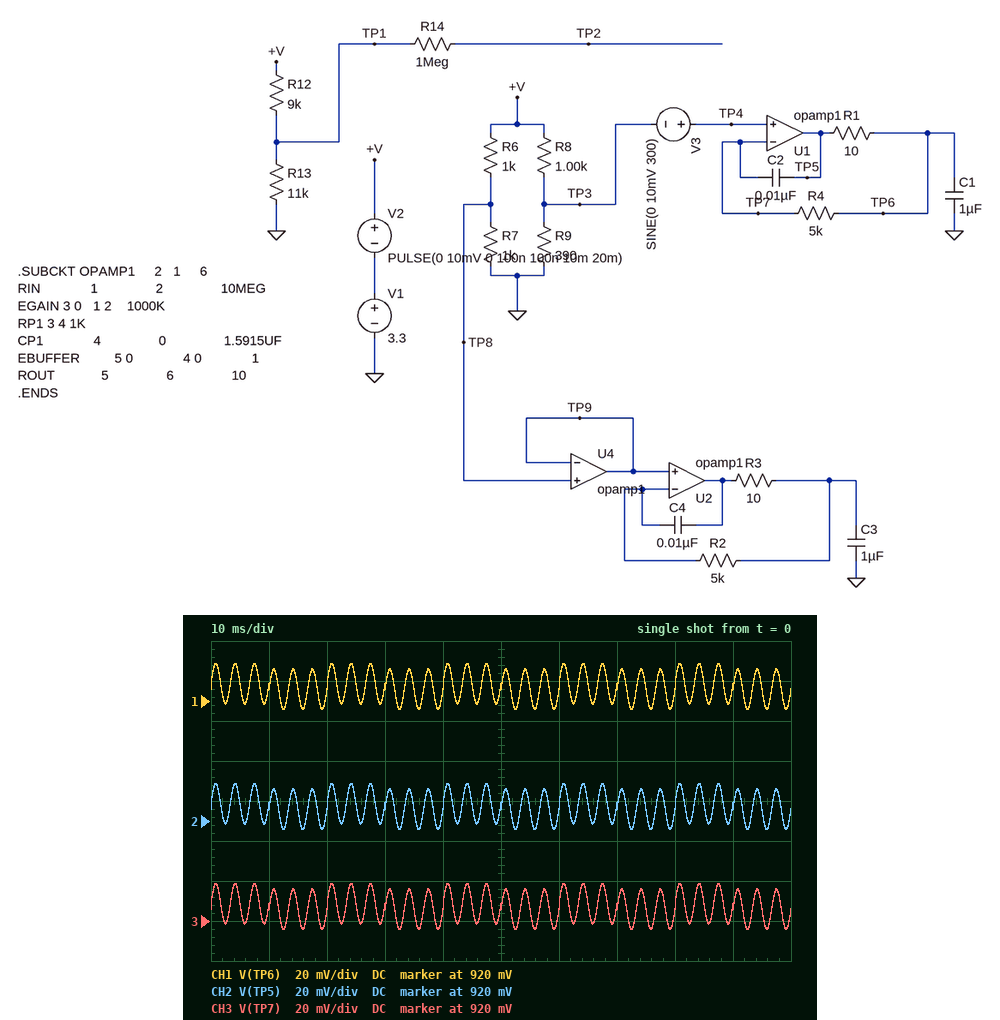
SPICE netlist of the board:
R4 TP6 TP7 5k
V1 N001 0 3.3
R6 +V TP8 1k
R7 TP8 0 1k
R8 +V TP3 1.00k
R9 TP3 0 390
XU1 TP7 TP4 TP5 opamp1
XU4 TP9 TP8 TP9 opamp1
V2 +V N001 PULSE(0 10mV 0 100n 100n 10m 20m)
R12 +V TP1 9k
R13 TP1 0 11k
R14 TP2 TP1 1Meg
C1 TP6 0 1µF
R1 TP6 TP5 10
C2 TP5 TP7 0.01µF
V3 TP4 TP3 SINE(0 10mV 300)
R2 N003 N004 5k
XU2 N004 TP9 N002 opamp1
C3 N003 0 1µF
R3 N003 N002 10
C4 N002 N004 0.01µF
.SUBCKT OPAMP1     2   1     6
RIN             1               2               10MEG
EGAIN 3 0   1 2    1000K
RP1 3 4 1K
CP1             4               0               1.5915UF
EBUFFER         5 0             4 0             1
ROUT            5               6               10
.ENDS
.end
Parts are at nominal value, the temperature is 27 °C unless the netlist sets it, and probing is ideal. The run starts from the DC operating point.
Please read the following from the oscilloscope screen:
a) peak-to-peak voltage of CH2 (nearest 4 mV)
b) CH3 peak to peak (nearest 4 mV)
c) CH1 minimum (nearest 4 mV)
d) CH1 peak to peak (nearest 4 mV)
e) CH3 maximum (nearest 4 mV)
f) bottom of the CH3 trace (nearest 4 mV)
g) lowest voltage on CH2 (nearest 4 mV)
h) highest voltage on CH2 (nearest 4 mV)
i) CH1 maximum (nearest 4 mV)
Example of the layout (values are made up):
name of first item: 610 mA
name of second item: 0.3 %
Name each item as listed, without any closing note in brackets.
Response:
peak-to-peak voltage of CH2: 24 mV
CH3 peak to peak: 24 mV
CH1 minimum: 916 mV
CH1 peak to peak: 24 mV
CH3 maximum: 940 mV
bottom of the CH3 trace: 916 mV
lowest voltage on CH2: 916 mV
highest voltage on CH2: 940 mV
CH1 maximum: 940 mV
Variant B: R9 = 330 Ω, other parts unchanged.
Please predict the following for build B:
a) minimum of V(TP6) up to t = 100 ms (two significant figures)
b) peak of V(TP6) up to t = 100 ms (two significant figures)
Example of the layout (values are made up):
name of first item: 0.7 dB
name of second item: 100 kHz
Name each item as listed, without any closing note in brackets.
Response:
minimum of V(TP6) up to t = 100 ms: 810 mV
peak of V(TP6) up to t = 100 ms: 830 mV
